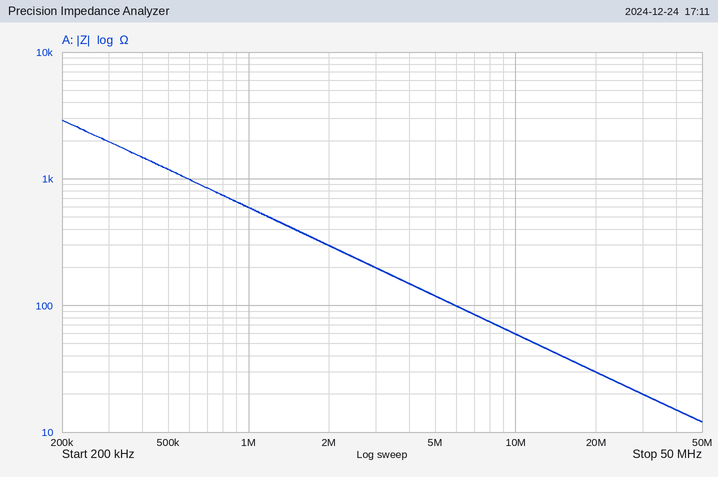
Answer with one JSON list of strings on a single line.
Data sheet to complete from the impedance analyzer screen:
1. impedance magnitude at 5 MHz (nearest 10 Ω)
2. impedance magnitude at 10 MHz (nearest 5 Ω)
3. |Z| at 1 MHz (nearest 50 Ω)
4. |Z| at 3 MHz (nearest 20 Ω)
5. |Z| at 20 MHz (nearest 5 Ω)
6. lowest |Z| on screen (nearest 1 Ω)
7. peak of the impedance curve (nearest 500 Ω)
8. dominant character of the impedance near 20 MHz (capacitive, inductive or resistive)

["120 Ω", "60 Ω", "600 Ω", "200 Ω", "30 Ω", "12 Ω", "3.0 kΩ", "capacitive"]
